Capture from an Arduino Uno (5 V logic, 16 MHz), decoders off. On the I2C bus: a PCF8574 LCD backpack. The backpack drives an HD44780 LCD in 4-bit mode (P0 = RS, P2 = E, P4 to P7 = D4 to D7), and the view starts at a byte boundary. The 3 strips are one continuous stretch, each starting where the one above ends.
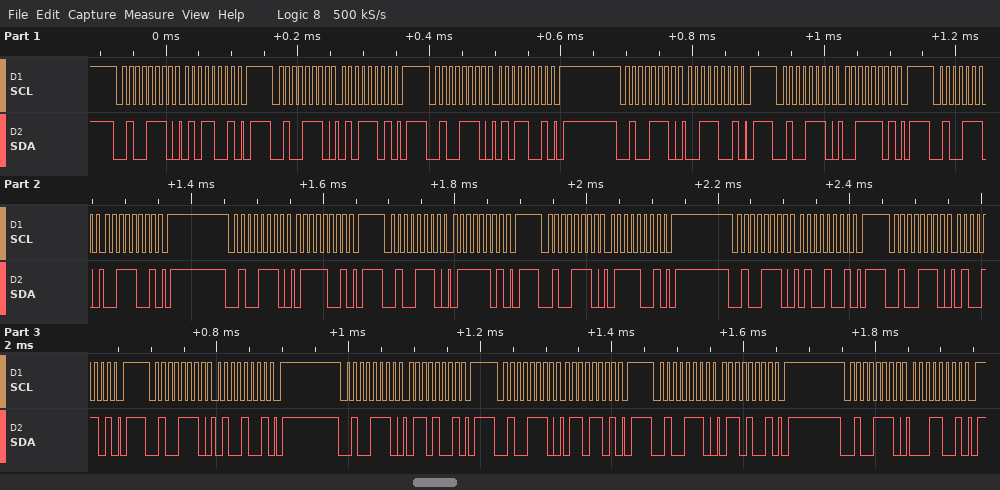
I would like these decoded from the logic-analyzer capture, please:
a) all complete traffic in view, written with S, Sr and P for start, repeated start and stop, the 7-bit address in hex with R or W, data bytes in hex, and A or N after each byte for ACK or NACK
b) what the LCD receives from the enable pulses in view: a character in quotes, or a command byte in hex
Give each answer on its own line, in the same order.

S 27W A 59 A P S 27W A 5D A P S 27W A 59 A P S 27W A 39 A P S 27W A 3D A P S 27W A 39 A P S 27W A 79 A P S 27W A 7D A P S 27W A 79 A P S 27W A 49 A P S 27W A 4D A P S 27W A 49 A P S 27W A 69 A P S 27W A 6D A P S 27W A 69 A P S 27W A 19 A P
'S' 't'
